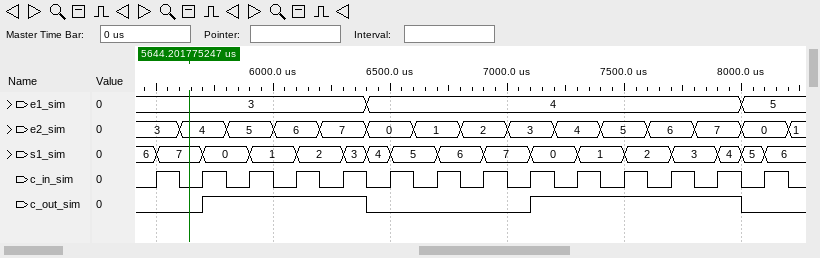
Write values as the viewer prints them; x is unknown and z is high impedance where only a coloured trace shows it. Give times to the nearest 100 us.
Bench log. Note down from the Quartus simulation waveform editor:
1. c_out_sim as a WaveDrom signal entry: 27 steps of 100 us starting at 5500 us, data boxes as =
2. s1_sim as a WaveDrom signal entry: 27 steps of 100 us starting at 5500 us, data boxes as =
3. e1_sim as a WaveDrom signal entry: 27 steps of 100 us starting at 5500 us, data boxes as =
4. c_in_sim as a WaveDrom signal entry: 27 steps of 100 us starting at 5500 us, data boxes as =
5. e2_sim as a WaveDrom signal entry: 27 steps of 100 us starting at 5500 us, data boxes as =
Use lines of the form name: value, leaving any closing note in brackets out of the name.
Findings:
c_out_sim as a WaveDrom signal entry: 27 steps of 100 us starting at 5500 us, data boxes as =: {name: 'c_out_sim', wave: '0.1......0......1........0.'}
s1_sim as a WaveDrom signal entry: 27 steps of 100 us starting at 5500 us, data boxes as =: {name: 's1_sim', wave: '=.=.=.=.===.=.=.=.=.=.=.===', data: '7 0 1 2 3 4 5 6 7 0 1 2 3 4 5 6'}
e1_sim as a WaveDrom signal entry: 27 steps of 100 us starting at 5500 us, data boxes as =: {name: 'e1_sim', wave: '=........=...............=.', data: '3 4 5'}
c_in_sim as a WaveDrom signal entry: 27 steps of 100 us starting at 5500 us, data boxes as =: {name: 'c_in_sim', wave: '101010101010101010101010101'}
e2_sim as a WaveDrom signal entry: 27 steps of 100 us starting at 5500 us, data boxes as =: {name: 'e2_sim', wave: '==.=.=.=.=.=.=.=.=.=.=.=.=.', data: '3 4 5 6 7 0 1 2 3 4 5 6 7 0'}
